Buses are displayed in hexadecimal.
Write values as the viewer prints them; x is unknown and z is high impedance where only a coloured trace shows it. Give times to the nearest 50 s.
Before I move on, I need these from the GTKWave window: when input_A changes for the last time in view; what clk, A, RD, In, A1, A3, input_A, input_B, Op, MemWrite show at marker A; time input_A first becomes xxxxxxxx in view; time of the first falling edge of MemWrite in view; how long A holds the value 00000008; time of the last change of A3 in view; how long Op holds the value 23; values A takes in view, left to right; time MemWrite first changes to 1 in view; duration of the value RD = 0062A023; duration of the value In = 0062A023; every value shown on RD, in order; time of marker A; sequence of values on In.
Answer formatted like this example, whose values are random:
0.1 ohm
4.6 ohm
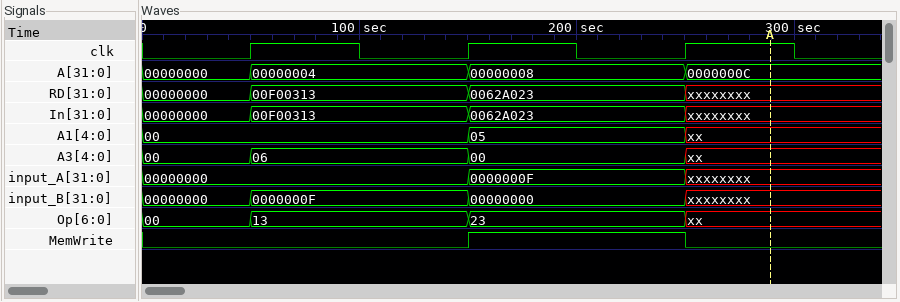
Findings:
250 s
clk=1, A=0000000C, RD=xxxxxxxx, In=xxxxxxxx, A1=xx, A3=xx, input_A=xxxxxxxx, input_B=xxxxxxxx, Op=xx, MemWrite=0
250 s
250 s
100 s
250 s
100 s
00000000, 00000004, 00000008, 0000000C
150 s
100 s
100 s
00000000, 00F00313, 0062A023, xxxxxxxx
300 s
00000000, 00F00313, 0062A023, xxxxxxxx
